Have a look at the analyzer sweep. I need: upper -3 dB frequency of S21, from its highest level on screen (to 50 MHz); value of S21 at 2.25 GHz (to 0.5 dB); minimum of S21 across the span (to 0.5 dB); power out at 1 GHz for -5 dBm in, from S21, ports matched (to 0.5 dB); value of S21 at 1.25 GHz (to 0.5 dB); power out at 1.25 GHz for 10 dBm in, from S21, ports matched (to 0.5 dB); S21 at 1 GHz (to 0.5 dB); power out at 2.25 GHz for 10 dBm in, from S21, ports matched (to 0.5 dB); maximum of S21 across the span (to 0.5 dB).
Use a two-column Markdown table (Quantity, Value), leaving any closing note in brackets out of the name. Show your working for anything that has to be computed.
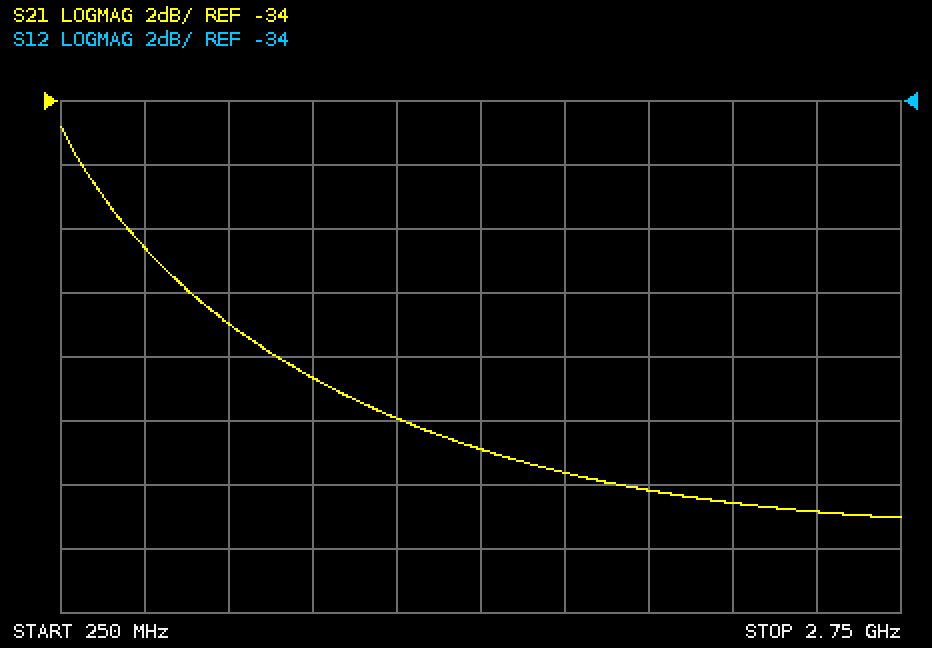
| Quantity | Value |
|---|---|
| upper -3 dB frequency of S21, from its highest level on screen | 450 MHz |
| value of S21 at 2.25 GHz | -46.5 dB |
| minimum of S21 across the span | -47.0 dB |
| power out at 1 GHz for -5 dBm in, from S21, ports matched | -5 dBm + (-42.5 dB) = -47.5 dBm |
| value of S21 at 1.25 GHz | -44.0 dB |
| power out at 1.25 GHz for 10 dBm in, from S21, ports matched | 10 dBm + (-44.0 dB) = -34.0 dBm |
| S21 at 1 GHz | -42.5 dB |
| power out at 2.25 GHz for 10 dBm in, from S21, ports matched | 10 dBm + (-46.5 dB) = -36.5 dBm |
| maximum of S21 across the span | -35.0 dB |
